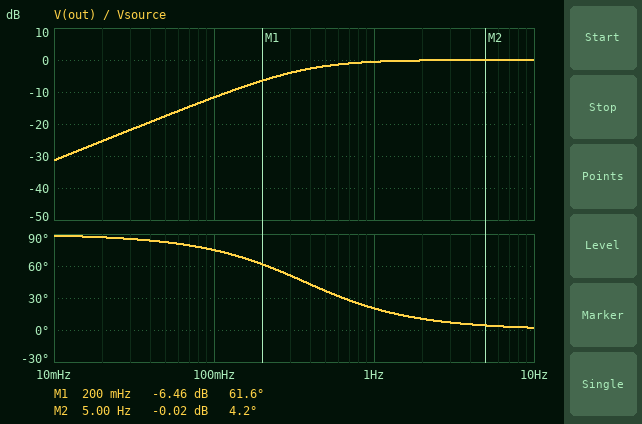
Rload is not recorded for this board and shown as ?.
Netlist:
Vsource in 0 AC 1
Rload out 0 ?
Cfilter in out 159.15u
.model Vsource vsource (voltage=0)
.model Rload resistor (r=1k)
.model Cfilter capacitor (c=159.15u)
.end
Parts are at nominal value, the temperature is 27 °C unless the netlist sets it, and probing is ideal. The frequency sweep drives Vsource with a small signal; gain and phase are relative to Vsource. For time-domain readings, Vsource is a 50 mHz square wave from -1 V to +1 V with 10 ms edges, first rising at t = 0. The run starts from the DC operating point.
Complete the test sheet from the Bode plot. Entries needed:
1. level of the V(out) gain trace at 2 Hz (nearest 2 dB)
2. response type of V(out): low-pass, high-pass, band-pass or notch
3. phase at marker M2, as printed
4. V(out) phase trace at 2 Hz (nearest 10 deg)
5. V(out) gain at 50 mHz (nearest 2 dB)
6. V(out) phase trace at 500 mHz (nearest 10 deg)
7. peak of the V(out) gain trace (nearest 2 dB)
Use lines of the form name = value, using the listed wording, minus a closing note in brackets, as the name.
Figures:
level of the V(out) gain trace at 2 Hz = 0 dB
response type of V(out): low-pass, high-pass, band-pass or notch = high-pass
phase at marker M2, as printed = 4.2 deg
V(out) phase trace at 2 Hz = 10 deg
V(out) gain at 50 mHz = -18 dB
V(out) phase trace at 500 mHz = 40 deg
peak of the V(out) gain trace = 0 dB
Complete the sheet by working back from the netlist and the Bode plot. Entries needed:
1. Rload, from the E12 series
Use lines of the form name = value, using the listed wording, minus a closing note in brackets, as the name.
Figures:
Rload, from the E12 series = 2.7 kΩ
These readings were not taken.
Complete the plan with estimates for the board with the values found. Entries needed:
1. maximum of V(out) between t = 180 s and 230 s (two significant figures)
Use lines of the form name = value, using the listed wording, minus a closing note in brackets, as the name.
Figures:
maximum of V(out) between t = 180 s and 230 s = 2.0 V
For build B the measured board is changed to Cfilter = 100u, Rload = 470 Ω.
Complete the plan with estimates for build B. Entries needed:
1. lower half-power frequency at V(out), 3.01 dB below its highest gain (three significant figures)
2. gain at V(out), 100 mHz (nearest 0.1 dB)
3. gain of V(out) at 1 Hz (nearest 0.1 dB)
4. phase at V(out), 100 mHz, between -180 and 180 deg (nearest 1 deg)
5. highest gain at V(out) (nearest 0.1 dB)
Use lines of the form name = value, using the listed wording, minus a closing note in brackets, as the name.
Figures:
lower half-power frequency at V(out), 3.01 dB below its highest gain = 3.39 Hz
gain at V(out), 100 mHz = -30.6 dB
gain of V(out) at 1 Hz = -11.0 dB
phase at V(out), 100 mHz, between -180 and 180 deg = 88 deg
highest gain at V(out) = 0 dB
